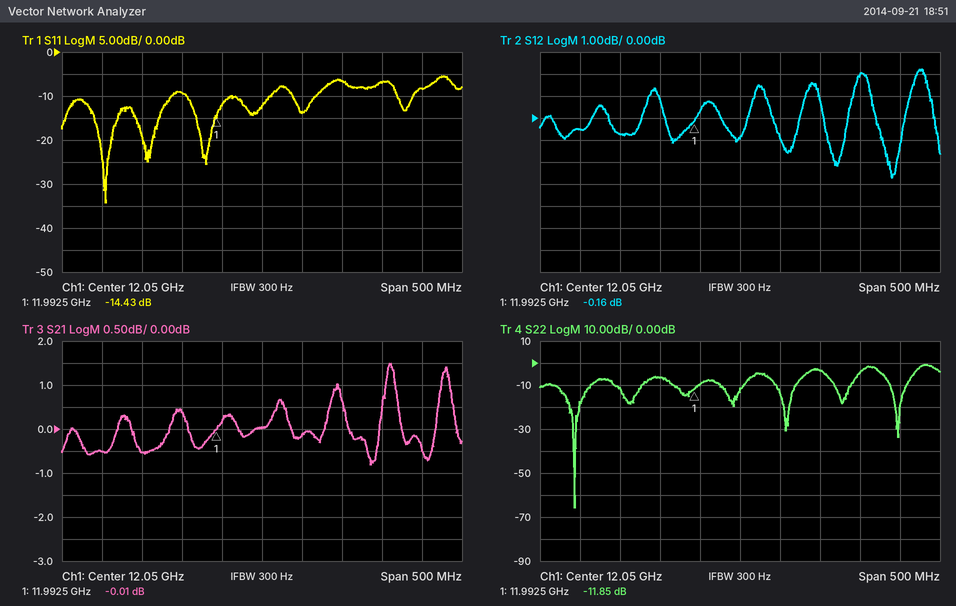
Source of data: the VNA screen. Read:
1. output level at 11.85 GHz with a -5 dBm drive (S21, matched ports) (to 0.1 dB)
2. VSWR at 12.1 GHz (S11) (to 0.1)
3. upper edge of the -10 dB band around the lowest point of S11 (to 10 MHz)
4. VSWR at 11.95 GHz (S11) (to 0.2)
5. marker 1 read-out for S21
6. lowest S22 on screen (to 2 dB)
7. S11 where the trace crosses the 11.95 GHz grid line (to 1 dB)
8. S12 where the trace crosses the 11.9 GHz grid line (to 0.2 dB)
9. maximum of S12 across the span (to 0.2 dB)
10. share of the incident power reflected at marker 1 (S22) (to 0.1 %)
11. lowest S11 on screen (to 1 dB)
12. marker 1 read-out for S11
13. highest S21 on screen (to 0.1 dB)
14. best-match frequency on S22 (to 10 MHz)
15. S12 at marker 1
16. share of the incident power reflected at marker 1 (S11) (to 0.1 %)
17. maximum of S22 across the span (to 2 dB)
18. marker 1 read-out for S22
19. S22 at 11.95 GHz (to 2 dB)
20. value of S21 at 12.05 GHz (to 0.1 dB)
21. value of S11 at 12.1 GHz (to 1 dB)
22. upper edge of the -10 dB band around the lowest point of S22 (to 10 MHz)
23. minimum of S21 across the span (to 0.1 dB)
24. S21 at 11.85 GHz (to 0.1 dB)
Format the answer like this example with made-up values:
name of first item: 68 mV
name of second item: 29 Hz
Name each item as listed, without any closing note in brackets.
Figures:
output level at 11.85 GHz with a -5 dBm drive (S21, matched ports): -5.5 dBm
VSWR at 12.1 GHz (S11): 1.5
upper edge of the -10 dB band around the lowest point of S11: 11.94 GHz
VSWR at 11.95 GHz (S11): 2.0
marker 1 read-out for S21: -0.01 dB
lowest S22 on screen: -66 dB
S11 where the trace crosses the 11.95 GHz grid line: -9 dB
S12 where the trace crosses the 11.9 GHz grid line: -0.8 dB
maximum of S12 across the span: 2.2 dB
share of the incident power reflected at marker 1 (S22): 6.5 %
lowest S11 on screen: -34 dB
marker 1 read-out for S11: -14.43 dB
highest S21 on screen: 1.5 dB
best-match frequency on S22: 11.84 GHz
S12 at marker 1: -0.16 dB
share of the incident power reflected at marker 1 (S11): 3.6 %
maximum of S22 across the span: 0 dB
marker 1 read-out for S22: -11.85 dB
S22 at 11.95 GHz: -6 dB
value of S21 at 12.05 GHz: 0.0 dB
value of S11 at 12.1 GHz: -14 dB
upper edge of the -10 dB band around the lowest point of S22: 11.86 GHz
minimum of S21 across the span: -0.8 dB
S21 at 11.85 GHz: -0.5 dB
